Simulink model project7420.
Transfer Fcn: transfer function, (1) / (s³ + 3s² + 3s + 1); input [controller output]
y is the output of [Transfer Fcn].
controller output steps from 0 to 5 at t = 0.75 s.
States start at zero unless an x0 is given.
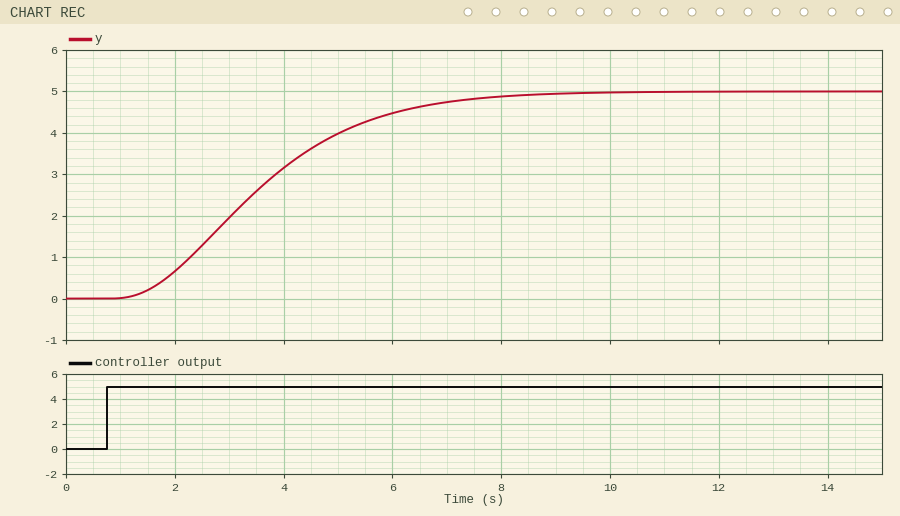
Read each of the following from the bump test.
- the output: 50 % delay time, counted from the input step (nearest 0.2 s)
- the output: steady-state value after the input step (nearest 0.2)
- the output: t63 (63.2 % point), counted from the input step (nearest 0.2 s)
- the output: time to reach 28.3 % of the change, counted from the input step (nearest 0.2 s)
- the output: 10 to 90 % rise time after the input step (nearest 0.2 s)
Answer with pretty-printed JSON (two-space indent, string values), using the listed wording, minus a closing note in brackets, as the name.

{
  "the output: 50 % delay time, counted from the input step": "2.6 s",
  "the output: steady-state value after the input step": "5.0",
  "the output: t63 (63.2 % point), counted from the input step": "3.2 s",
  "the output: time to reach 28.3 % of the change, counted from the input step": "1.8 s",
  "the output: 10 to 90 % rise time after the input step": "4.2 s"
}
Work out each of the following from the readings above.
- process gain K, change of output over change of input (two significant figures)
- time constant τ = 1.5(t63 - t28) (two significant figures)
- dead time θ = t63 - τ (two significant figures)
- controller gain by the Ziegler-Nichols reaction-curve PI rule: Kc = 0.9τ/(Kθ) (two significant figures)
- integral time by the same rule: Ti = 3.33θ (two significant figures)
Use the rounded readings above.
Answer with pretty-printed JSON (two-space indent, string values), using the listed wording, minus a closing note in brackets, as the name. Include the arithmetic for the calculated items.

{
  "process gain K, change of output over change of input": "(5 - 0) / 5 = 1.0",
  "time constant τ = 1.5(t63 - t28)": "1.5 × (3.2 - 1.8) = 2.1 s",
  "dead time θ = t63 - τ": "3.2 - 2.1 = 1.1 s",
  "controller gain by the Ziegler-Nichols reaction-curve PI rule: Kc = 0.9τ/(Kθ)": "0.9 × 2.1 / (1 × 1.1) = 1.7",
  "integral time by the same rule: Ti = 3.33θ": "3.33 × 1.1 = 3.7 s"
}
